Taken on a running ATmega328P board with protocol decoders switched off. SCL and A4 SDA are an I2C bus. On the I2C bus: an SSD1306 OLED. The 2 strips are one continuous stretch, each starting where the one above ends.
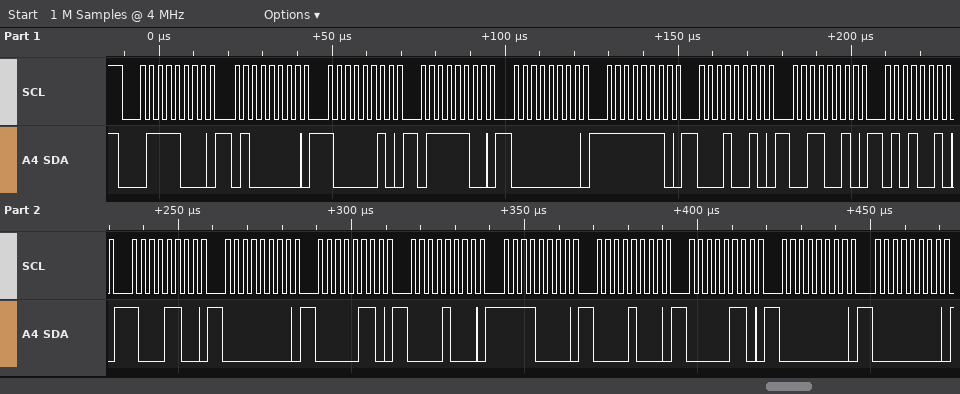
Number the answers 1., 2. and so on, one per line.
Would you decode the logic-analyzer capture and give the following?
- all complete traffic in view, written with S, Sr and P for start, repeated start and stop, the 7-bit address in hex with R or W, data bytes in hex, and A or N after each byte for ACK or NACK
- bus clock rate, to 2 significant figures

1. S 3CW A 40 A 82 A 7C A 00 A FE A 12 A 32 A 52 A 8C A 00 A 06 A 08 A F0 A 08 A 06 A 00 A 00 A
2. 400 kHz
